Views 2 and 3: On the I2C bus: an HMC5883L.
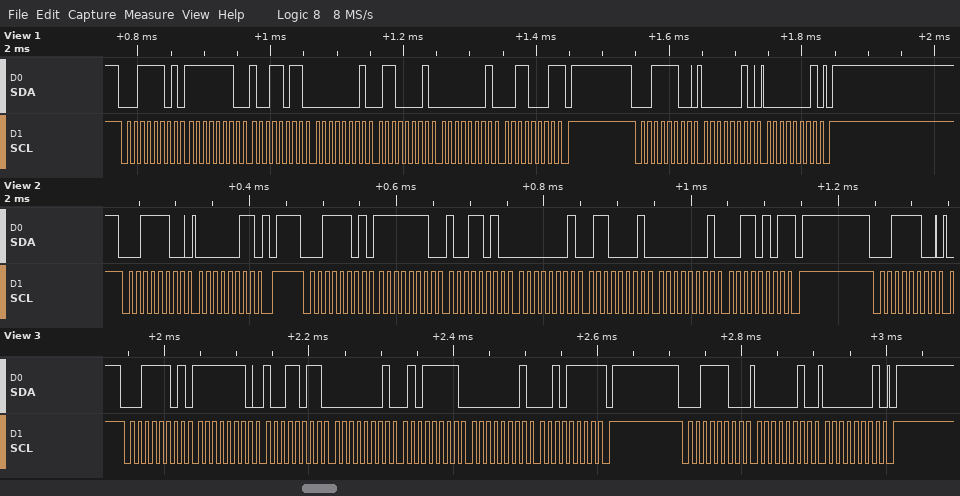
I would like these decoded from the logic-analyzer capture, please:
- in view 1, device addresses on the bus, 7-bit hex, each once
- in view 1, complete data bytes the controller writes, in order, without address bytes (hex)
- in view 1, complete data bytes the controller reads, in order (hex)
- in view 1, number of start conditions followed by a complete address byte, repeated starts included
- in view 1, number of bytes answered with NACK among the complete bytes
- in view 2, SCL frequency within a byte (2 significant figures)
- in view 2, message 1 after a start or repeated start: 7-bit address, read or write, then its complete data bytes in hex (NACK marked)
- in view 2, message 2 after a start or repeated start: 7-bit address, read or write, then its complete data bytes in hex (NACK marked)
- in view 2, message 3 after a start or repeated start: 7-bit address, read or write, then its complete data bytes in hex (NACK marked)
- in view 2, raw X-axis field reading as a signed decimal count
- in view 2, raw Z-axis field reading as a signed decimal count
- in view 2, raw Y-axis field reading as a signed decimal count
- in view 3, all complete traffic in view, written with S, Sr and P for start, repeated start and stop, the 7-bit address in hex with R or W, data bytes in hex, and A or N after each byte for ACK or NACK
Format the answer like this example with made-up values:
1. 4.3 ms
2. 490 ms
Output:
1. 0x1E
2. 02 01
3. FE 9B 01 61 01 31
4. 2
5. 1
6. 100 kHz
7. 0x1E write: 03
8. 0x1E read: FE 9A 01 61 01 35 NACK
9. 0x1E write
10. -358
11. 353
12. 309
13. S 1ER A FE A 9B A 01 A 5F A 01 A 2F N P S 1EW A 02 A 01 A P
